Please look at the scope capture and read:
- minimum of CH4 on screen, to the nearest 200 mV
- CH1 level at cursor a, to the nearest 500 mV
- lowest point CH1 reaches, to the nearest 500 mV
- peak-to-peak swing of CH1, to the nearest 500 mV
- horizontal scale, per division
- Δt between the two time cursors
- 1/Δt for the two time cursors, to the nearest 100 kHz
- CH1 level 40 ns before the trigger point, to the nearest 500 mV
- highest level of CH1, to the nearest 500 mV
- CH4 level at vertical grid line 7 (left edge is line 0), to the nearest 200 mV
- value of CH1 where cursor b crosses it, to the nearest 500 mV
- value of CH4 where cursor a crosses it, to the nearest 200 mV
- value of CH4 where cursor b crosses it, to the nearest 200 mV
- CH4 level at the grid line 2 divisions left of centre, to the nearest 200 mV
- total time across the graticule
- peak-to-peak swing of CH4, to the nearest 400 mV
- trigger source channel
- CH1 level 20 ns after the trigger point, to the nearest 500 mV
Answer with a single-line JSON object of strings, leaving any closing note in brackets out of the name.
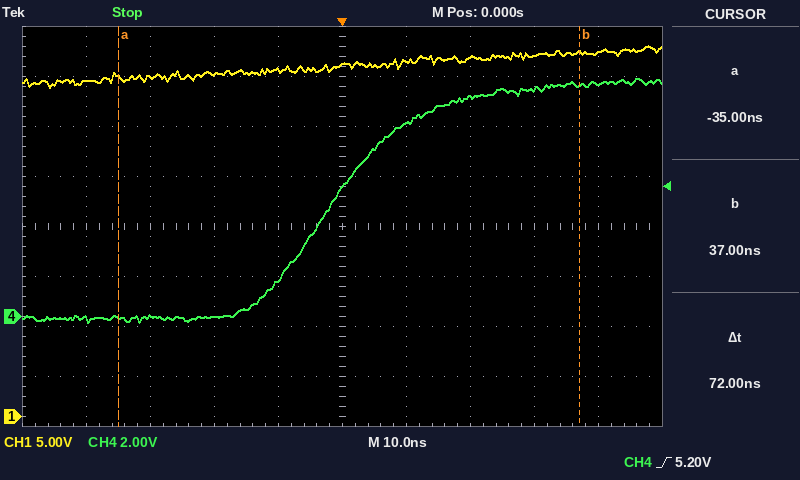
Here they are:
{"minimum of CH4 on screen, to the nearest 200 mV": "-200 mV", "CH1 level at cursor a, to the nearest 500 mV": "34.0 V", "lowest point CH1 reaches, to the nearest 500 mV": "33.0 V", "peak-to-peak swing of CH1, to the nearest 500 mV": "4.0 V", "horizontal scale, per division": "10 ns", "Δt between the two time cursors": "72 ns", "1/Δt for the two time cursors, to the nearest 100 kHz": "13.9 MHz", "CH1 level 40 ns before the trigger point, to the nearest 500 mV": "33.5 V", "highest level of CH1, to the nearest 500 mV": "37.0 V", "CH4 level at vertical grid line 7 (left edge is line 0), to the nearest 200 mV": "8.8 V", "value of CH1 where cursor b crosses it, to the nearest 500 mV": "36.5 V", "value of CH4 where cursor a crosses it, to the nearest 200 mV": "0.0 V", "value of CH4 where cursor b crosses it, to the nearest 200 mV": "9.2 V", "CH4 level at the grid line 2 divisions left of centre, to the nearest 200 mV": "0.0 V", "total time across the graticule": "100 ns", "peak-to-peak swing of CH4, to the nearest 400 mV": "9.6 V", "trigger source channel": "CH4", "CH1 level 20 ns after the trigger point, to the nearest 500 mV": "36.0 V"}
